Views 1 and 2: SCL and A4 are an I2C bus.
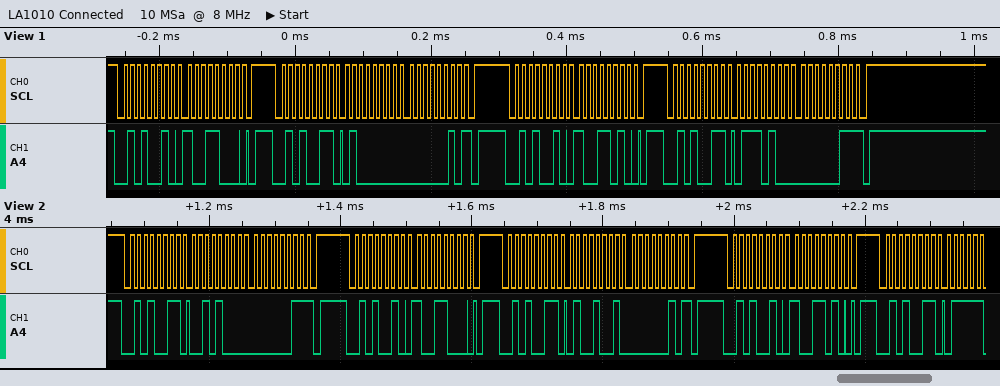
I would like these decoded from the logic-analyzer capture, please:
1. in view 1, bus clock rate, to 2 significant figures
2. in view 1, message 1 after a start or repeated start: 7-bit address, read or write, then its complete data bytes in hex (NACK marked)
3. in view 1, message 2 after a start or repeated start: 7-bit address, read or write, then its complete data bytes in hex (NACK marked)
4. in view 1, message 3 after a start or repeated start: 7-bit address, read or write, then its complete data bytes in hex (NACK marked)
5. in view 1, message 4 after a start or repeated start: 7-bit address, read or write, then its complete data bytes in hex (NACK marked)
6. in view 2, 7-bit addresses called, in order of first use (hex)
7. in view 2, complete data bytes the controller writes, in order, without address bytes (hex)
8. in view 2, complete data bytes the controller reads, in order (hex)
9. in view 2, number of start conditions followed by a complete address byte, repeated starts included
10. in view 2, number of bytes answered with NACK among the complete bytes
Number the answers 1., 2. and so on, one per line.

1. 100 kHz
2. 0x29 write: 98
3. 0x29 read: 40 02 NACK
4. 0x29 write: 9A
5. 0x29 read: 74 03 NACK
6. 0x29
7. 98 9A
8. 28 03 49 02
9. 5
10. 2
